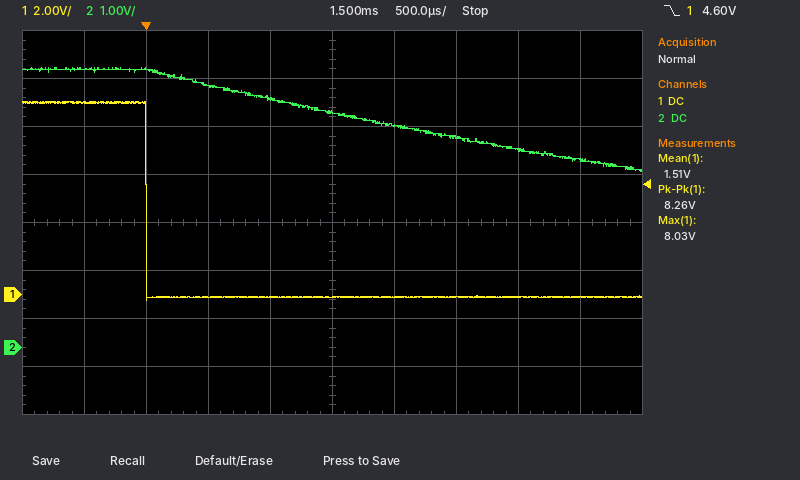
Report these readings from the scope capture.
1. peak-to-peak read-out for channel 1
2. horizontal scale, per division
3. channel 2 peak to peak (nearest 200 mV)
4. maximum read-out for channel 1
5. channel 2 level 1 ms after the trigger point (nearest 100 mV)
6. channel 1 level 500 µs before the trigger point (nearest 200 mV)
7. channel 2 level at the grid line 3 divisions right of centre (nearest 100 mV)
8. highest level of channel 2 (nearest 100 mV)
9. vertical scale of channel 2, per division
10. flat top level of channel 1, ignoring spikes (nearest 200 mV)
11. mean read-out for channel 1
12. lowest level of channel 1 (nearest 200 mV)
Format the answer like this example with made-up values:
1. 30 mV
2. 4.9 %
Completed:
1. 8.26 V
2. 500 µs
3. 2.2 V
4. 8.03 V
5. 5.2 V
6. 8.0 V
7. 4.1 V
8. 5.8 V
9. 1 V
10. 8.0 V
11. 1.51 V
12. -200 mV
